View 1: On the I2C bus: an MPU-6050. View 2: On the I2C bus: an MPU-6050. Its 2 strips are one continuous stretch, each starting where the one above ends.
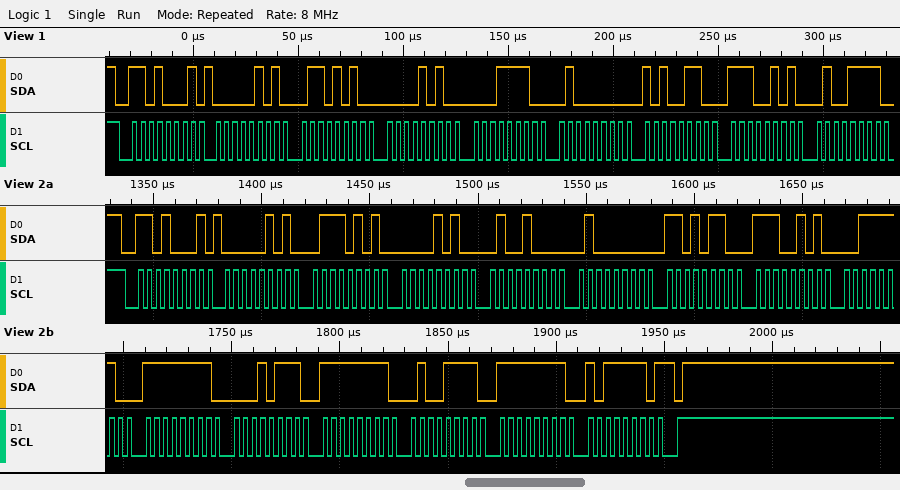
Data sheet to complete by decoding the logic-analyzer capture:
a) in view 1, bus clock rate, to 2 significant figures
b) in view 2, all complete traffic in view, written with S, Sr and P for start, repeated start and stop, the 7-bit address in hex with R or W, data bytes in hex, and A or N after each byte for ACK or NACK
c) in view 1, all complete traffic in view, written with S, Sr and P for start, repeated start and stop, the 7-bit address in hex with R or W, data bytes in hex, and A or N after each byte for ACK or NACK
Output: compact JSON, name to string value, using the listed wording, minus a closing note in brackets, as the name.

{"in view 1, bus clock rate, to 2 significant figures": "250 kHz", "in view 2, all complete traffic in view, written with S, Sr and P for start, repeated start and stop, the 7-bit address in hex with R or W, data bytes in hex, and A or N after each byte for ACK or NACK": "S 68R A 05 A 75 A 0A A 48 A 40 A D6 A E5 A 3E A FF A 17 A FF A 4F A FF A BE N P", "in view 1, all complete traffic in view, written with S, Sr and P for start, repeated start and stop, the 7-bit address in hex with R or W, data bytes in hex, and A or N after each byte for ACK or NACK": "S 68R A 05 A 6A A 0A A 1E A 40 A A6 A E5 A 4F A"}
